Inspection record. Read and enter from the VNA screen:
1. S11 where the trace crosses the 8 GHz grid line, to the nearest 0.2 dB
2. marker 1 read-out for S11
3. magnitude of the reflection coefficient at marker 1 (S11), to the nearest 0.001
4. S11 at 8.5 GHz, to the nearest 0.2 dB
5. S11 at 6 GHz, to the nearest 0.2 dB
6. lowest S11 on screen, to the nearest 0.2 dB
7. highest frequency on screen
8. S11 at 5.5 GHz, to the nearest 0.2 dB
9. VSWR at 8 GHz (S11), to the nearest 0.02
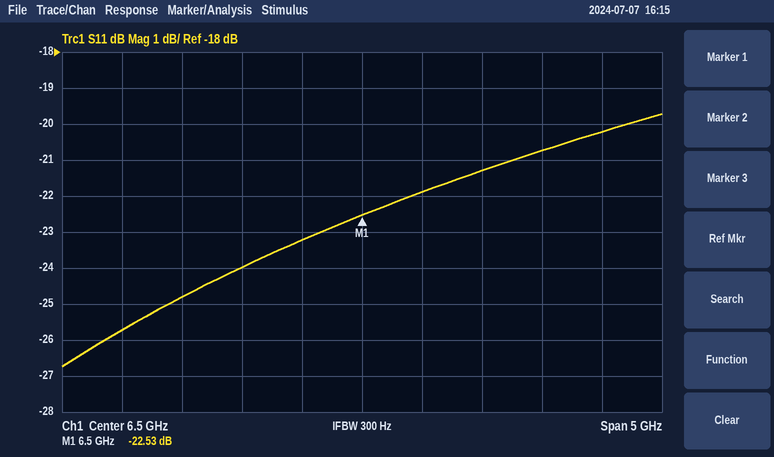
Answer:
-20.8 dB
-22.53 dB
0.075
-20.2 dB
-23.2 dB
-26.8 dB
9 GHz
-24.0 dB
1.20
